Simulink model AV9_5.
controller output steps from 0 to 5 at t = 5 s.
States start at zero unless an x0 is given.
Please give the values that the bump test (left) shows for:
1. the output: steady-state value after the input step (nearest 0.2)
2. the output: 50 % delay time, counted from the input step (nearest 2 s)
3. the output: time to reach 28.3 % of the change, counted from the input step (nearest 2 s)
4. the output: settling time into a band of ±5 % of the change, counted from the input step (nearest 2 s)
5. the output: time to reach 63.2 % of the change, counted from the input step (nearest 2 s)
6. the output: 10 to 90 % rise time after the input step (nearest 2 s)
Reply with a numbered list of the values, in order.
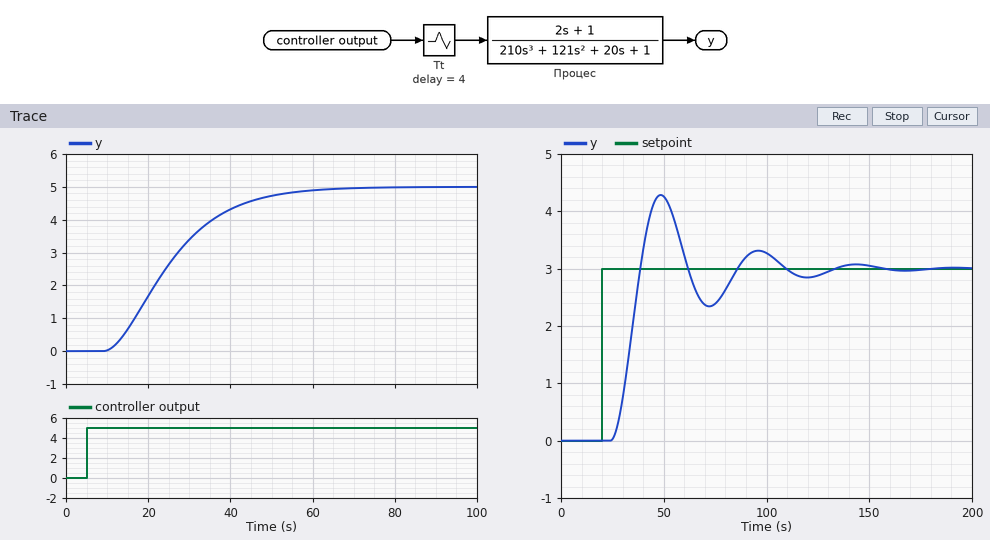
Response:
1. 5.0
2. 20 s
3. 14 s
4. 46 s
5. 24 s
6. 30 s
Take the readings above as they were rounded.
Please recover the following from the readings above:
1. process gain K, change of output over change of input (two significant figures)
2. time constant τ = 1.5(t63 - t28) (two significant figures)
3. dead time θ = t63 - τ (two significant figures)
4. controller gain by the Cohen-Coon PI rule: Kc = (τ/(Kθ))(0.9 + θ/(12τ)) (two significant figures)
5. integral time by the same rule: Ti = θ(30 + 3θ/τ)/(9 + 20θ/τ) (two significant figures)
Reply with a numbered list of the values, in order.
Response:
1. 1.0
2. 15 s
3. 9.0 s
4. 1.6
5. 14 s
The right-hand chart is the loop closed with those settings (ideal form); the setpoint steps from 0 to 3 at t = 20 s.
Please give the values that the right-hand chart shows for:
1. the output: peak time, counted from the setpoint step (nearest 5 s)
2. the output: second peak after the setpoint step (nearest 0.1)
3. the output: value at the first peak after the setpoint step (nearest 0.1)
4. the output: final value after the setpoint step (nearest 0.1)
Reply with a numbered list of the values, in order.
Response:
1. 30 s
2. 3.3
3. 4.3
4. 3.0
